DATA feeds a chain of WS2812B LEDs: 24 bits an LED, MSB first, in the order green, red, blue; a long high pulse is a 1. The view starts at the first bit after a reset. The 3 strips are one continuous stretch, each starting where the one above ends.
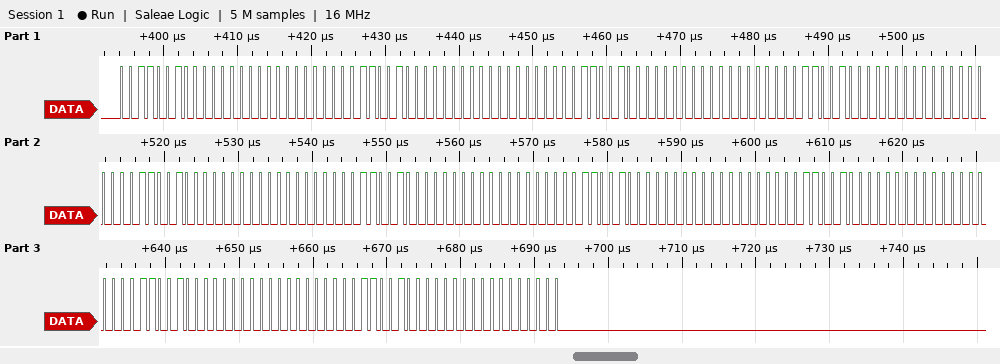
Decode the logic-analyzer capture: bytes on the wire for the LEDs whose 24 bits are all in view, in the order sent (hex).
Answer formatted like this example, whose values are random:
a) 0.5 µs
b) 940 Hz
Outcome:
a) 32 00 00 32 00 00 32 00 00 32 00 00 32 00 00 32 00 00 32 00 00 32 00 00 32 00 00 32 00 00
